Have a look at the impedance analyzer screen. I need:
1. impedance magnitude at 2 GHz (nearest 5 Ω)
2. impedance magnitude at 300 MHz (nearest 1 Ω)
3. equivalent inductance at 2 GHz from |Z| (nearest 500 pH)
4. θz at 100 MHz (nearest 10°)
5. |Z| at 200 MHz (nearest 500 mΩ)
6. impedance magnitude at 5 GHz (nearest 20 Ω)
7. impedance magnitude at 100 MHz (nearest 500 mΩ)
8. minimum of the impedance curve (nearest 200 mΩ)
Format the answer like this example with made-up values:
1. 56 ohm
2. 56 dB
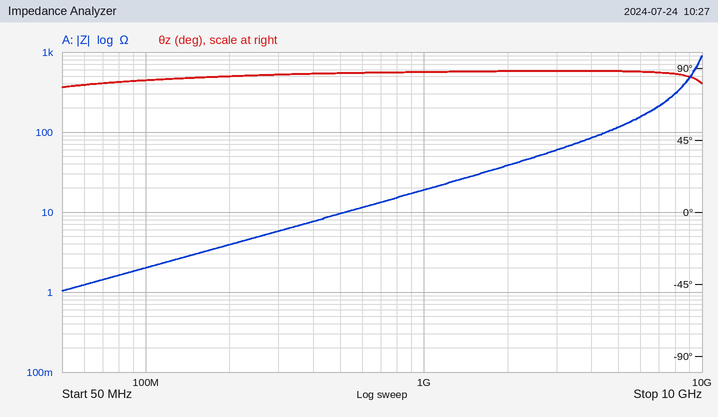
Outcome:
1. 40 Ω
2. 6 Ω
3. 3.0 nH
4. 80°
5. 4.0 Ω
6. 120 Ω
7. 2.0 Ω
8. 1.0 Ω
